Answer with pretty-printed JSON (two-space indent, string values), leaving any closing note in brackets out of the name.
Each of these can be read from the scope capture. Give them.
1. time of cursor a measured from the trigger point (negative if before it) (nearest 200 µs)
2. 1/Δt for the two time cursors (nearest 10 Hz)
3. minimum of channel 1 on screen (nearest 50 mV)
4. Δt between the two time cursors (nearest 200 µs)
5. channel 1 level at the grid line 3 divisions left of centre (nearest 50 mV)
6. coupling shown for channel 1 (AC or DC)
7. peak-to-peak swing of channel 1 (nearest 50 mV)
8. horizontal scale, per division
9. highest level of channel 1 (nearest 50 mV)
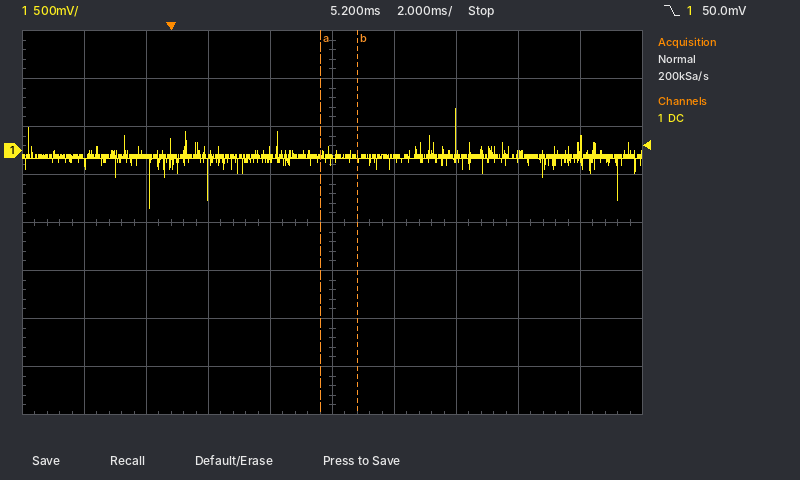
{
  "time of cursor a measured from the trigger point (negative if before it)": "+4.8 ms",
  "1/Δt for the two time cursors": "830 Hz",
  "minimum of channel 1 on screen": "-600 mV",
  "Δt between the two time cursors": "1.2 ms",
  "channel 1 level at the grid line 3 divisions left of centre": "-50 mV",
  "coupling shown for channel 1": "DC",
  "peak-to-peak swing of channel 1": "1.05 V",
  "horizontal scale, per division": "2 ms",
  "highest level of channel 1": "450 mV"
}
